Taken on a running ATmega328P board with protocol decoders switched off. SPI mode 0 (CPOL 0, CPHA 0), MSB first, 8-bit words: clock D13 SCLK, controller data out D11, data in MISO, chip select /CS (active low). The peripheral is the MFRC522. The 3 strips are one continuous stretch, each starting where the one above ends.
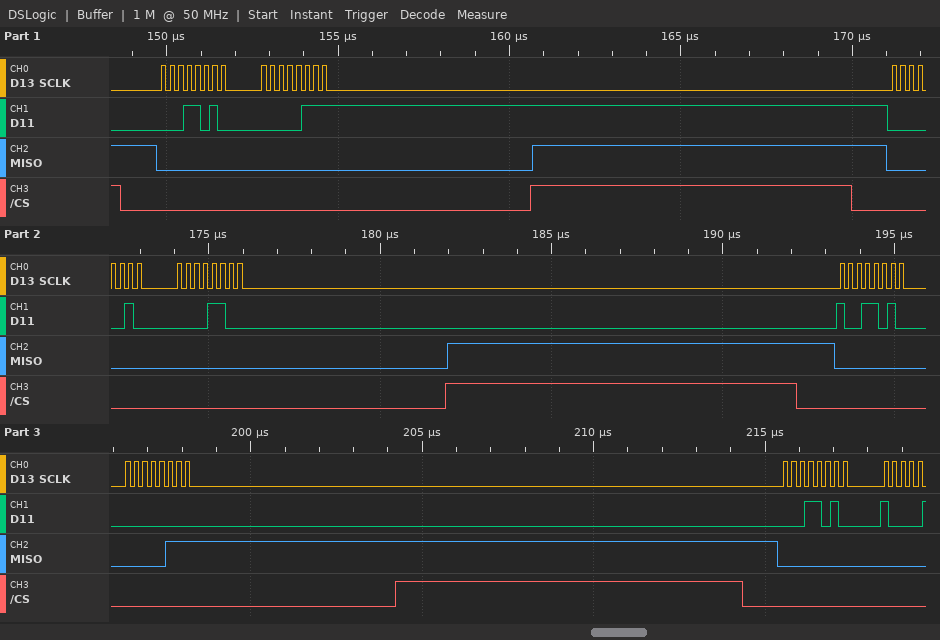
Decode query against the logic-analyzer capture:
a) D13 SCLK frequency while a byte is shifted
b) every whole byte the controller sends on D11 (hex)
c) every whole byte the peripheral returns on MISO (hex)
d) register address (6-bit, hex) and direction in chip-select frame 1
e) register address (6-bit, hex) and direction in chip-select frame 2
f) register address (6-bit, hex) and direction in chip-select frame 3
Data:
4 MHz
0x1A 0x07 0x02 0x0C 0x9A 0x00 0x1A
0x00 0x00 0x00 0x00 0x00 0x07 0x00
0x0D write
0x01 write
0x0D read
